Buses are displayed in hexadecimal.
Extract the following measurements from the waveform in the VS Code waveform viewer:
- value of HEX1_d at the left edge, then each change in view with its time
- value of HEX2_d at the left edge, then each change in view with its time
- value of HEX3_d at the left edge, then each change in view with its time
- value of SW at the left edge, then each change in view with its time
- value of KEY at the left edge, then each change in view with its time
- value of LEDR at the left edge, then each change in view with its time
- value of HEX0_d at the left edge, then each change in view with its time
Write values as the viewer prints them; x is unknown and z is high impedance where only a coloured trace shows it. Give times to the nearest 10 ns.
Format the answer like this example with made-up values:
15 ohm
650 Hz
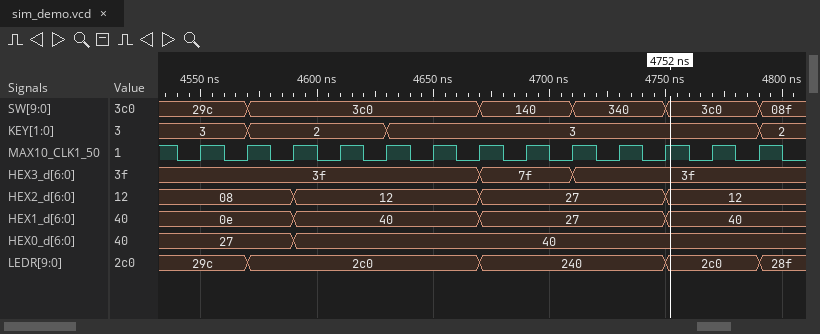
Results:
0e, 40 at 4590 ns, 27 at 4670 ns, 40 at 4750 ns
08, 12 at 4590 ns, 27 at 4670 ns, 12 at 4750 ns
3f, 7f at 4670 ns, 3f at 4710 ns
29c, 3c0 at 4570 ns, 140 at 4670 ns, 340 at 4710 ns, 3c0 at 4750 ns, 08f at 4790 ns
3, 2 at 4570 ns, 3 at 4630 ns, 2 at 4790 ns
29c, 2c0 at 4570 ns, 240 at 4670 ns, 2c0 at 4750 ns, 28f at 4790 ns
27, 40 at 4590 ns
